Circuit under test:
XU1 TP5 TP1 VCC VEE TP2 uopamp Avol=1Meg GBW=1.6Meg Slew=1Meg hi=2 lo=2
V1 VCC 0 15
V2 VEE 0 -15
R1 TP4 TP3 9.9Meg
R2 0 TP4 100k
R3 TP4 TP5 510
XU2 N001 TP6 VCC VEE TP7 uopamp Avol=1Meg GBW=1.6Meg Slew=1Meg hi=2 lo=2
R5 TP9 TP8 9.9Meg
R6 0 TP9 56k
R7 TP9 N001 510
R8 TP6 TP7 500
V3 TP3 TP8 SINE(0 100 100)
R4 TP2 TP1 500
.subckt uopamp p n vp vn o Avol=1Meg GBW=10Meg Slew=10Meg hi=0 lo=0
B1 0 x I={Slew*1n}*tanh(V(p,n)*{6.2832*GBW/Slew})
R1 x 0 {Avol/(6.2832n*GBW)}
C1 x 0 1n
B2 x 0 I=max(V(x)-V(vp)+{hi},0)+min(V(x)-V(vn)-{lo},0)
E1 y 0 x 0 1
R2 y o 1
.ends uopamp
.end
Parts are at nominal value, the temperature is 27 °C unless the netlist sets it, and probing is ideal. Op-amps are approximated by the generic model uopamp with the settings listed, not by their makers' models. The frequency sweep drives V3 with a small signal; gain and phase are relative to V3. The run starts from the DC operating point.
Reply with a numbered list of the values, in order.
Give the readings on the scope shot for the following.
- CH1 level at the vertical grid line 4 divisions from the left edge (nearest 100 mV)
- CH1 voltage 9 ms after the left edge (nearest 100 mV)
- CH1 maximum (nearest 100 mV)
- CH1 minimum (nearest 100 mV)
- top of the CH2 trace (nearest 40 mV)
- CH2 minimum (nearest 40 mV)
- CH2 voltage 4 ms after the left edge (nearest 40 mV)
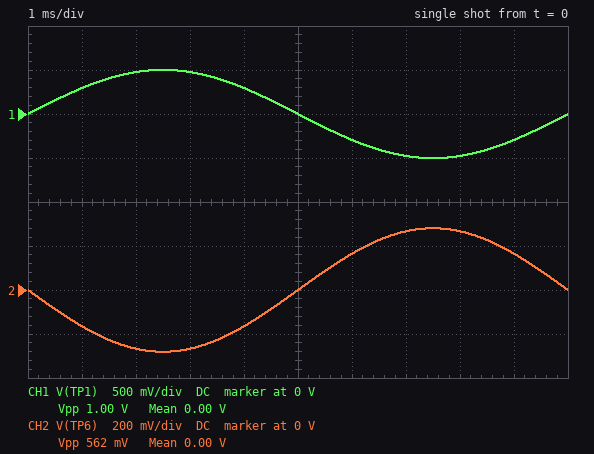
1. 300 mV
2. -300 mV
3. 500 mV
4. -500 mV
5. 280 mV
6. -280 mV
7. -160 mV
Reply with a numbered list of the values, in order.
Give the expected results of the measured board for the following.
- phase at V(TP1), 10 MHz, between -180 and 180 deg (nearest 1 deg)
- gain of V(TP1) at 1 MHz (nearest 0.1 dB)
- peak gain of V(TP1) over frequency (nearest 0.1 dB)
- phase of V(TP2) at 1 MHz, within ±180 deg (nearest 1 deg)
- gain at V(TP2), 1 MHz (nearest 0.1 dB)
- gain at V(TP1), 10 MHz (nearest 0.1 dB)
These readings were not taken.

1. -81 deg
2. -47.4 dB
3. -46.0 dB
4. -32 deg
5. -47.4 dB
6. -62.0 dB
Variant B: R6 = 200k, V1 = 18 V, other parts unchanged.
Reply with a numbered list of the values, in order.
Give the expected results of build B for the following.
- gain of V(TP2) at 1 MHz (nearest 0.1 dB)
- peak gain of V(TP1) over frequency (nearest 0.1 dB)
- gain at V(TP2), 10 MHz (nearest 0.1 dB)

1. -47.5 dB
2. -46.1 dB
3. -62.1 dB
